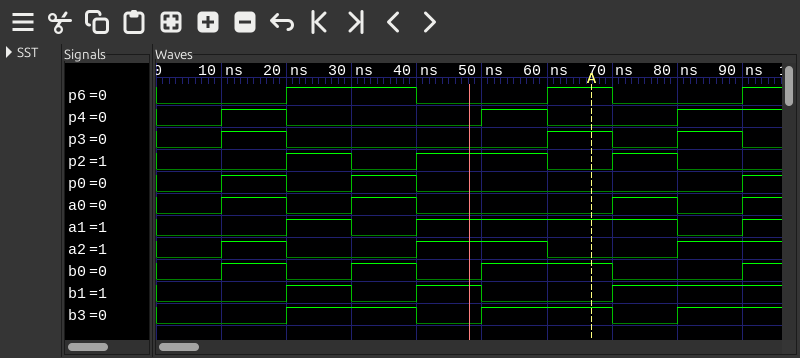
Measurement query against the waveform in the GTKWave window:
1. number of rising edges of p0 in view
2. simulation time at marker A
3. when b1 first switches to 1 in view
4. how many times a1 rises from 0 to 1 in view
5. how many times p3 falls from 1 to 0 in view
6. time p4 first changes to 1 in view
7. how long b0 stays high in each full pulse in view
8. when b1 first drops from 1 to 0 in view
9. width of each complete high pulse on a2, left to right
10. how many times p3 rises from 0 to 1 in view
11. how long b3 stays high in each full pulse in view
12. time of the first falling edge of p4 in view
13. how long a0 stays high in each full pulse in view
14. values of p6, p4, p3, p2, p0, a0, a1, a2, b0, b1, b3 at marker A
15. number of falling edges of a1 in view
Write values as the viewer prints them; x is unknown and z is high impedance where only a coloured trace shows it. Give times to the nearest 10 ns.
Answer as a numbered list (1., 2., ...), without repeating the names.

1. 3
2. 70 ns
3. 20 ns
4. 3
5. 3
6. 10 ns
7. 10 ns, 10 ns, 20 ns
8. 30 ns
9. 10 ns, 20 ns
10. 3
11. 20 ns, 20 ns
12. 20 ns
13. 10 ns, 10 ns, 10 ns
14. p6=1, p4=0, p3=1, p2=0, p0=0, a0=0, a1=1, a2=0, b0=1, b1=0, b3=1
15. 2
